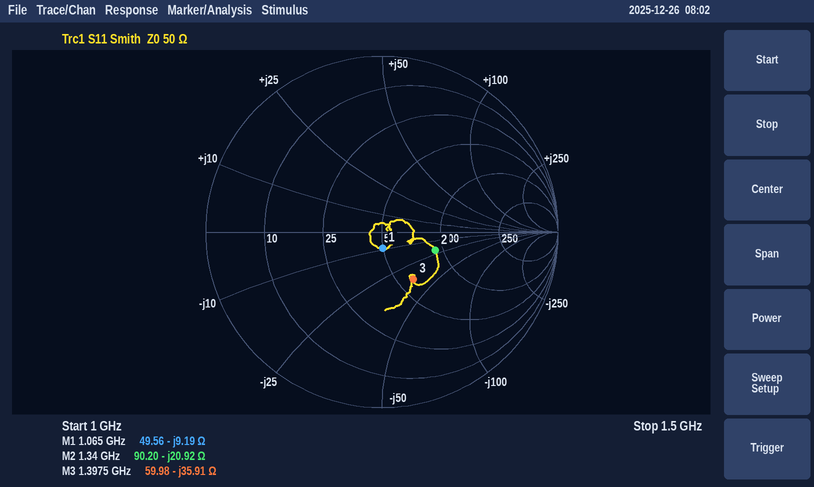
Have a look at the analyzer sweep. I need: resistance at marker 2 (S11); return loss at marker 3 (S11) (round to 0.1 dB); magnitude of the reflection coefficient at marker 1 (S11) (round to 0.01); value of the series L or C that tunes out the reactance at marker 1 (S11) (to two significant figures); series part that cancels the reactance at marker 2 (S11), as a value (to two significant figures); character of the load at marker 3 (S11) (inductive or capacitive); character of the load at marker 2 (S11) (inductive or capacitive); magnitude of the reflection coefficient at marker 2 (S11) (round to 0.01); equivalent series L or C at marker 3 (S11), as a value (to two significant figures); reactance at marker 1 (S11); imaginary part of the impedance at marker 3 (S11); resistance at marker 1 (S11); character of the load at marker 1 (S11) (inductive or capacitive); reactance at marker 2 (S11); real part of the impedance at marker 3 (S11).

90.20 Ω
9.8 dB
0.09
1.4 nH
2.5 nH
capacitive
capacitive
0.32
3.2 pF
-9.19 Ω
-35.91 Ω
49.56 Ω
capacitive
-20.92 Ω
59.98 Ω
